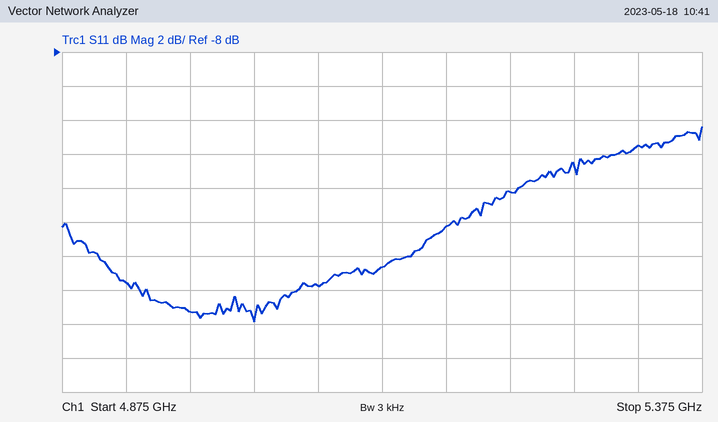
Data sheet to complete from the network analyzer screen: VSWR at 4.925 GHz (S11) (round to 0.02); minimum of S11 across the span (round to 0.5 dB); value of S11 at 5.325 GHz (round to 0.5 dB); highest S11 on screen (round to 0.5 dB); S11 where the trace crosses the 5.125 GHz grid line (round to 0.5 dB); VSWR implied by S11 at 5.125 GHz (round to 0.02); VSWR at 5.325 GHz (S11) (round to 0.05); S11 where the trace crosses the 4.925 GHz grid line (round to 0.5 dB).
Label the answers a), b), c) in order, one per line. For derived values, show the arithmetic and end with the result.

a) |Γ| = 10^(-21.5/20) = 0.0841; VSWR = (1 + 0.0841)/(1 − 0.0841) ≈ 1.18
b) -24.0 dB
c) -13.5 dB
d) -12.5 dB
e) -20.5 dB
f) |Γ| = 10^(-20.5/20) = 0.0944; VSWR = (1 + 0.0944)/(1 − 0.0944) ≈ 1.21, so 1.20 to the nearest 0.02
g) |Γ| = 10^(-13.5/20) = 0.2113; VSWR = (1 + 0.2113)/(1 − 0.2113) ≈ 1.54, so 1.55 to the nearest 0.05
h) -21.5 dB
